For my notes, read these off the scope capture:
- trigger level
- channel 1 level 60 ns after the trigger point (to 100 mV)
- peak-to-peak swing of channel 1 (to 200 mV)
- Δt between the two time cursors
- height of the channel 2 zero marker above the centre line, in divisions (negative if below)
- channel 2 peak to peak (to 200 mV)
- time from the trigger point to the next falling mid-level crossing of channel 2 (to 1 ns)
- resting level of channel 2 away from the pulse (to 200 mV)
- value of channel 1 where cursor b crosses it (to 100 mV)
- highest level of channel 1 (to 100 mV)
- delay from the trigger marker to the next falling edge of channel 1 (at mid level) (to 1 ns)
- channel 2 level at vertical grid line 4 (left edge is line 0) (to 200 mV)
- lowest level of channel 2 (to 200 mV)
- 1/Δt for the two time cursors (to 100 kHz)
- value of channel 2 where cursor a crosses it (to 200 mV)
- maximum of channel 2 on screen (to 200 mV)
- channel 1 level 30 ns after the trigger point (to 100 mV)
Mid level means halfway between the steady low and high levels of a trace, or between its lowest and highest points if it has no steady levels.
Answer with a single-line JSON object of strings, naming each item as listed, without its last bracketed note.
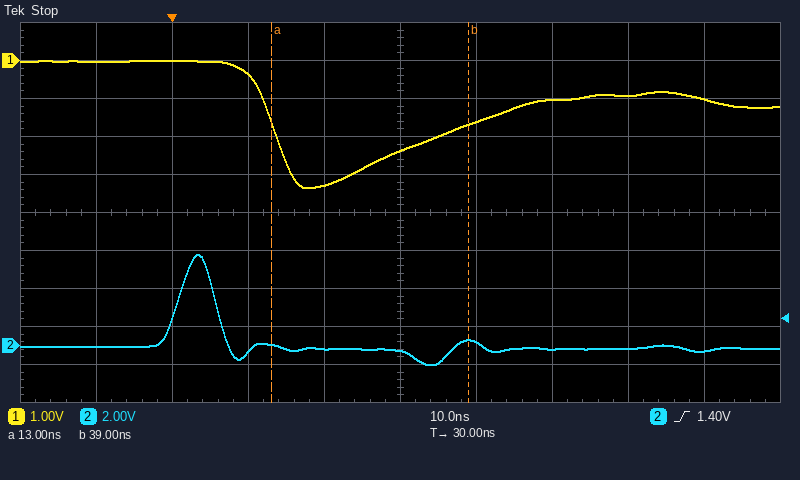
{"trigger level": "1.40 V", "channel 1 level 60 ns after the trigger point": "-900 mV", "peak-to-peak swing of channel 1": "3.4 V", "Δt between the two time cursors": "26 ns", "height of the channel 2 zero marker above the centre line, in divisions": "-3.5 div", "channel 2 peak to peak": "5.8 V", "time from the trigger point to the next falling mid-level crossing of channel 2": "6 ns", "resting level of channel 2 away from the pulse": "-200 mV", "value of channel 1 where cursor b crosses it": "-1.7 V", "highest level of channel 1": "0.0 V", "delay from the trigger marker to the next falling edge of channel 1 (at mid level)": "13 ns", "channel 2 level at vertical grid line 4 (left edge is line 0)": "-200 mV", "lowest level of channel 2": "-1.0 V", "1/Δt for the two time cursors": "38.5 MHz", "value of channel 2 where cursor a crosses it": "0.0 V", "maximum of channel 2 on screen": "4.8 V", "channel 1 level 30 ns after the trigger point": "-2.4 V"}
